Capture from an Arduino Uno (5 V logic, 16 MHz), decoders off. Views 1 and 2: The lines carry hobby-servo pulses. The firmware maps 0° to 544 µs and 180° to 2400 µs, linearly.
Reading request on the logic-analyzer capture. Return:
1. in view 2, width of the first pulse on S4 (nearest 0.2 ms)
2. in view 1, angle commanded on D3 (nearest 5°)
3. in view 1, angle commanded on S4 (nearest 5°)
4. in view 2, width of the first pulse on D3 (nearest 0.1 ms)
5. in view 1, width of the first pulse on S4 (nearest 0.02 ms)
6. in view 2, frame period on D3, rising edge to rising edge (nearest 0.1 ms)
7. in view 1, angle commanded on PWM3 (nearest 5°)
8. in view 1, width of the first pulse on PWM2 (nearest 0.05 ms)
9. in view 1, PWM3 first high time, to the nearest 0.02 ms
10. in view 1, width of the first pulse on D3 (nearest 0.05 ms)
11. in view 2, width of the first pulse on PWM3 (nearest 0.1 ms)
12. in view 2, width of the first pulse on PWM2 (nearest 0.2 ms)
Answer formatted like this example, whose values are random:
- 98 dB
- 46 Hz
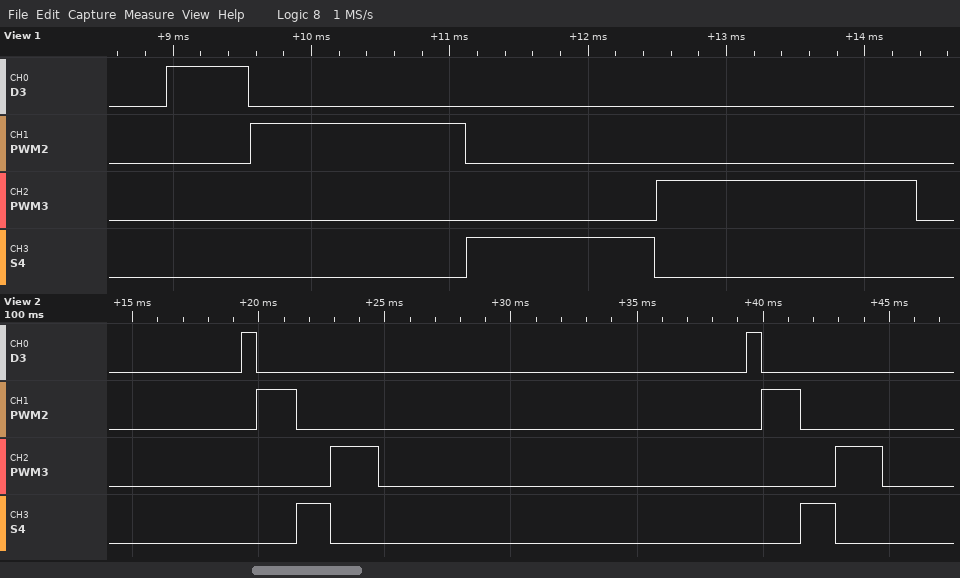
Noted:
- 1.4 ms
- 5°
- 80°
- 0.6 ms
- 1.36 ms
- 20.0 ms
- 130°
- 1.55 ms
- 1.88 ms
- 0.60 ms
- 1.9 ms
- 1.6 ms
